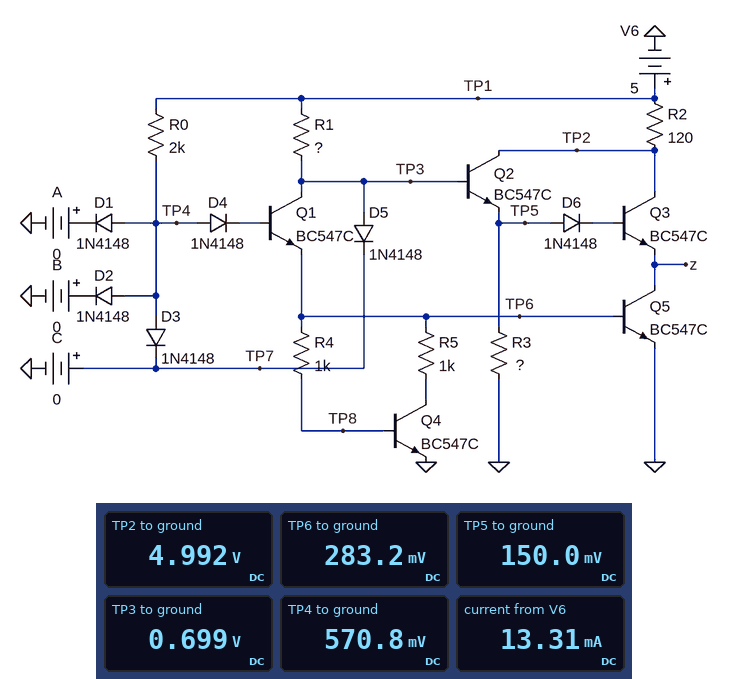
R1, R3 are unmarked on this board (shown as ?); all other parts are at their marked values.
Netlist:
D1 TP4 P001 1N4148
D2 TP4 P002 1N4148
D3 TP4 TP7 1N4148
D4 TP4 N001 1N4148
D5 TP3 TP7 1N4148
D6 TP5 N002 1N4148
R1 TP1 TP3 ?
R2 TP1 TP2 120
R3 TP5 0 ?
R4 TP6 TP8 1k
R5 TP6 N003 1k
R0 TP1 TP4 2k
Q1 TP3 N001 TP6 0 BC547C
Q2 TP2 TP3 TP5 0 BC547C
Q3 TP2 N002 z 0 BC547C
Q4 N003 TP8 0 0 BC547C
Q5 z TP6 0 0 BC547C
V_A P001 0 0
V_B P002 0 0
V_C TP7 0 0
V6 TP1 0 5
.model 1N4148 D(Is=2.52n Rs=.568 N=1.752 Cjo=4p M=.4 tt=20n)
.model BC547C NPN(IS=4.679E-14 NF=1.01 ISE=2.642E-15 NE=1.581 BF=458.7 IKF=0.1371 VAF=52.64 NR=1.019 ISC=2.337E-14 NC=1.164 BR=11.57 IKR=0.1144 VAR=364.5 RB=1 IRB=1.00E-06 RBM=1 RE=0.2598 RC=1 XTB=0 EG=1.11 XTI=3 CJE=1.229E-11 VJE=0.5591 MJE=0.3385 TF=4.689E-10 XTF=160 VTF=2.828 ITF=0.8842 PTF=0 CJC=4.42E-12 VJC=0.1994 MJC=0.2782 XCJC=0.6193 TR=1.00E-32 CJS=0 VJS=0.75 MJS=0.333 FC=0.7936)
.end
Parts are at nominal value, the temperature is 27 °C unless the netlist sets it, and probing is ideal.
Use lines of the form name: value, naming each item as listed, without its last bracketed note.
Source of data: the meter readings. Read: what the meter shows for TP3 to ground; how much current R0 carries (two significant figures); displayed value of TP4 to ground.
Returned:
what the meter shows for TP3 to ground: 0.699 V
how much current R0 carries: 2.2 mA
displayed value of TP4 to ground: 570.8 mV
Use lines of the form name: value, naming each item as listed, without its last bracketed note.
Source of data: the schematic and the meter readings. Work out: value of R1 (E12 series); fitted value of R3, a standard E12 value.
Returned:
value of R1: 390 Ω
fitted value of R3, a standard E12 value: 2.2 kΩ
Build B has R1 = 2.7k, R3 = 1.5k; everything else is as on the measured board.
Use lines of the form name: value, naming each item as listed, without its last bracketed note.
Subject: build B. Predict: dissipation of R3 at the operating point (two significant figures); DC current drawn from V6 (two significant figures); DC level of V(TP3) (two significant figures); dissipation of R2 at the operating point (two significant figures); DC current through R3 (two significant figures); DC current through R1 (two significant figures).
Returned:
dissipation of R3 at the operating point: 3.1 µW
DC current drawn from V6: 3.9 mA
DC level of V(TP3): 610 mV
dissipation of R2 at the operating point: 250 nW
DC current through R3: 46 µA
DC current through R1: 1.6 mA
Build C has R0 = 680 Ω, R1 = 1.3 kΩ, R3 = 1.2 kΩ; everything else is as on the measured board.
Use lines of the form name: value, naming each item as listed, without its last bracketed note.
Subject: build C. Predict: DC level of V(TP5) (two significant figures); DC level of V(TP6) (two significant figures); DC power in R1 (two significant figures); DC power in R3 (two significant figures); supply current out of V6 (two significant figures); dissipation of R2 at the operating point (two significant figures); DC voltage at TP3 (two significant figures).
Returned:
DC level of V(TP5): 89 mV
DC level of V(TP6): 310 mV
DC power in R1: 15 mW
DC power in R3: 6.7 µW
supply current out of V6: 9.9 mA
dissipation of R2 at the operating point: 660 nW
DC voltage at TP3: 640 mV
